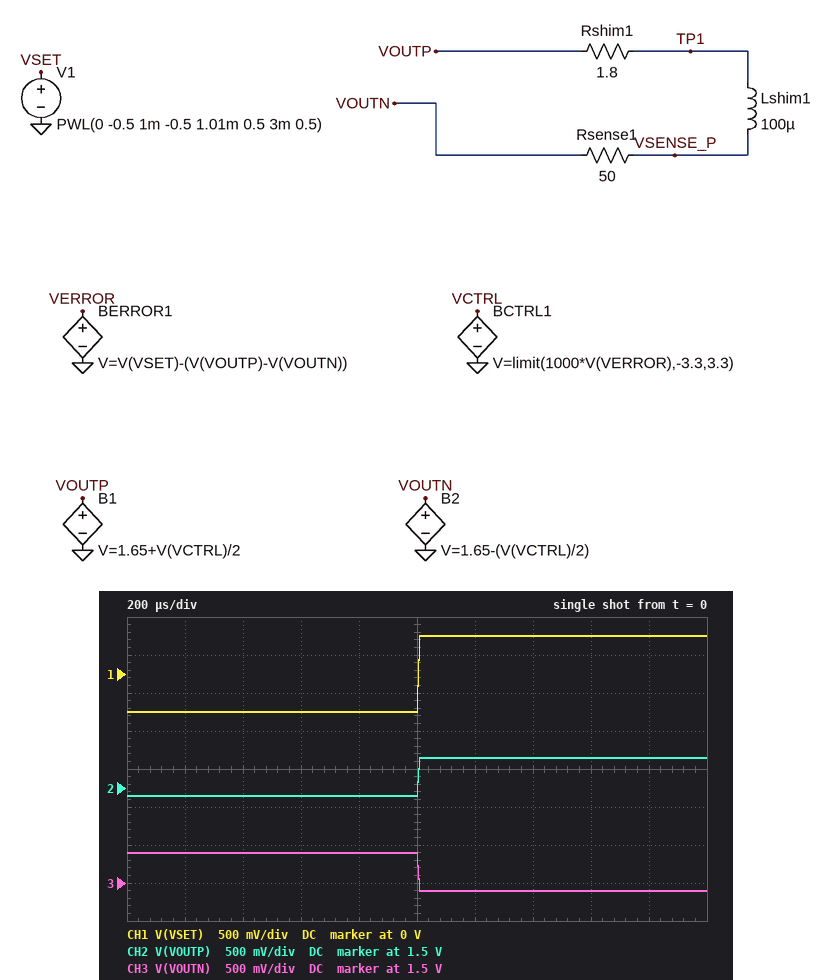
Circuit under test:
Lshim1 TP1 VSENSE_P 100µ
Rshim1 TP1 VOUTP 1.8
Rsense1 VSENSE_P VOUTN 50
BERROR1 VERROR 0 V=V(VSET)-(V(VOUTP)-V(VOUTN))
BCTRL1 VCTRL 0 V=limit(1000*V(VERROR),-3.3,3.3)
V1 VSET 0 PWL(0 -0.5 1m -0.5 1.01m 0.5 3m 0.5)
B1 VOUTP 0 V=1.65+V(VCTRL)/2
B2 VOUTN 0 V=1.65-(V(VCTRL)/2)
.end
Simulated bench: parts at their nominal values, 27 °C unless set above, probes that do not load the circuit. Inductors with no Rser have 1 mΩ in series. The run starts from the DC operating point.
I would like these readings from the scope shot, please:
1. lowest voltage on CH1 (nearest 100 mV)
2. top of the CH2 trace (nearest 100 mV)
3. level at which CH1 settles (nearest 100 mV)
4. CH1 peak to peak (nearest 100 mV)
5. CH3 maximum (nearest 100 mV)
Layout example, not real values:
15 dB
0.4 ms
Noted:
-500 mV
1.9 V
500 mV
1.0 V
1.9 V
